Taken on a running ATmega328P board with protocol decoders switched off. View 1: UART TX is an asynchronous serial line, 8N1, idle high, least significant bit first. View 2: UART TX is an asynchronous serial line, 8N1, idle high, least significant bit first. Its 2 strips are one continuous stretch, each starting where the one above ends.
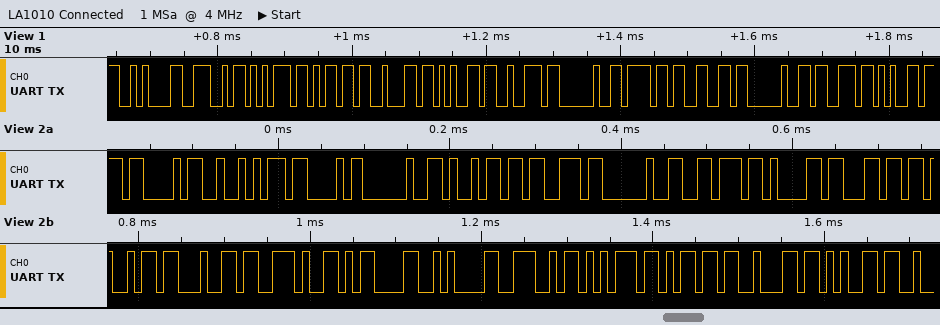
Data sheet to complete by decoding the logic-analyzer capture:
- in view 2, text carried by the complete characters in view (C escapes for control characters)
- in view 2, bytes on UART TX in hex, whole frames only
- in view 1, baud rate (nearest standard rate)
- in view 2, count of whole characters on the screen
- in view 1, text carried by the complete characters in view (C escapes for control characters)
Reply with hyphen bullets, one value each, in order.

- "CRC is valid.\r\nNumbe"
- 43 52 43 20 69 73 20 76 61 6C 69 64 2E 0D 0A 4E 75 6D 62 65
- 115200 baud
- 20
- "\nNumber of se"
